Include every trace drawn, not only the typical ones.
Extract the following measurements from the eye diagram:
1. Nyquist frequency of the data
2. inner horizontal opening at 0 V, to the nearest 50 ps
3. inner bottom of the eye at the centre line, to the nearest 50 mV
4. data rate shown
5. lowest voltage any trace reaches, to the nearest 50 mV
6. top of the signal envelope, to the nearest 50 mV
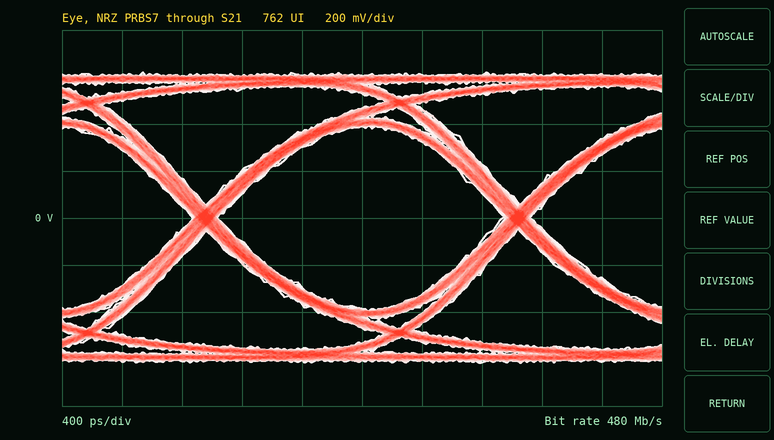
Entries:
240 MHz
1.90 ns
-400 mV
480 Mb/s
-600 mV
600 mV
